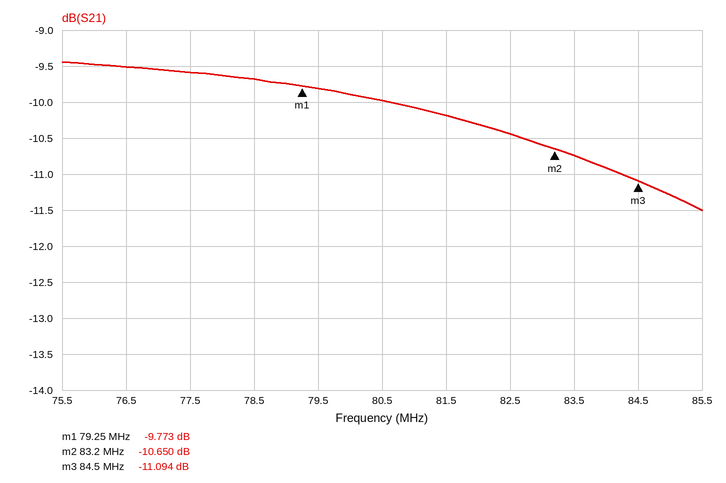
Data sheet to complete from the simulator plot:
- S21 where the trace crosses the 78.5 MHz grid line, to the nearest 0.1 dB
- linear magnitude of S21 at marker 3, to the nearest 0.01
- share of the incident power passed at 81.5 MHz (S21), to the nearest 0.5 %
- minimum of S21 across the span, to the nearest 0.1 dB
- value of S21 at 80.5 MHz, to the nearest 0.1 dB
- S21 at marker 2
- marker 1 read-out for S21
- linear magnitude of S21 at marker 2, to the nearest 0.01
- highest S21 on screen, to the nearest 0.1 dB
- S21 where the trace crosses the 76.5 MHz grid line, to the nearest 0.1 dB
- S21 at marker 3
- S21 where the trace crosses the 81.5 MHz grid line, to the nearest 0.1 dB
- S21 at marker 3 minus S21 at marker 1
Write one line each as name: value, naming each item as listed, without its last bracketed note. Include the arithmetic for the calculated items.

S21 where the trace crosses the 78.5 MHz grid line, to the nearest 0.1 dB: -9.7 dB
linear magnitude of S21 at marker 3, to the nearest 0.01: 10^(-11.094/20) ≈ 0.28
share of the incident power passed at 81.5 MHz (S21), to the nearest 0.5 %: 10^(-10.2/10) ≈ 9.5 %
minimum of S21 across the span, to the nearest 0.1 dB: -11.5 dB
value of S21 at 80.5 MHz, to the nearest 0.1 dB: -10.0 dB
S21 at marker 2: -10.650 dB
marker 1 read-out for S21: -9.773 dB
linear magnitude of S21 at marker 2, to the nearest 0.01: 10^(-10.65/20) ≈ 0.29
highest S21 on screen, to the nearest 0.1 dB: -9.4 dB
S21 where the trace crosses the 76.5 MHz grid line, to the nearest 0.1 dB: -9.5 dB
S21 at marker 3: -11.094 dB
S21 where the trace crosses the 81.5 MHz grid line, to the nearest 0.1 dB: -10.2 dB
S21 at marker 3 minus S21 at marker 1: -11.094 − (-9.773) = -1.321 dB
